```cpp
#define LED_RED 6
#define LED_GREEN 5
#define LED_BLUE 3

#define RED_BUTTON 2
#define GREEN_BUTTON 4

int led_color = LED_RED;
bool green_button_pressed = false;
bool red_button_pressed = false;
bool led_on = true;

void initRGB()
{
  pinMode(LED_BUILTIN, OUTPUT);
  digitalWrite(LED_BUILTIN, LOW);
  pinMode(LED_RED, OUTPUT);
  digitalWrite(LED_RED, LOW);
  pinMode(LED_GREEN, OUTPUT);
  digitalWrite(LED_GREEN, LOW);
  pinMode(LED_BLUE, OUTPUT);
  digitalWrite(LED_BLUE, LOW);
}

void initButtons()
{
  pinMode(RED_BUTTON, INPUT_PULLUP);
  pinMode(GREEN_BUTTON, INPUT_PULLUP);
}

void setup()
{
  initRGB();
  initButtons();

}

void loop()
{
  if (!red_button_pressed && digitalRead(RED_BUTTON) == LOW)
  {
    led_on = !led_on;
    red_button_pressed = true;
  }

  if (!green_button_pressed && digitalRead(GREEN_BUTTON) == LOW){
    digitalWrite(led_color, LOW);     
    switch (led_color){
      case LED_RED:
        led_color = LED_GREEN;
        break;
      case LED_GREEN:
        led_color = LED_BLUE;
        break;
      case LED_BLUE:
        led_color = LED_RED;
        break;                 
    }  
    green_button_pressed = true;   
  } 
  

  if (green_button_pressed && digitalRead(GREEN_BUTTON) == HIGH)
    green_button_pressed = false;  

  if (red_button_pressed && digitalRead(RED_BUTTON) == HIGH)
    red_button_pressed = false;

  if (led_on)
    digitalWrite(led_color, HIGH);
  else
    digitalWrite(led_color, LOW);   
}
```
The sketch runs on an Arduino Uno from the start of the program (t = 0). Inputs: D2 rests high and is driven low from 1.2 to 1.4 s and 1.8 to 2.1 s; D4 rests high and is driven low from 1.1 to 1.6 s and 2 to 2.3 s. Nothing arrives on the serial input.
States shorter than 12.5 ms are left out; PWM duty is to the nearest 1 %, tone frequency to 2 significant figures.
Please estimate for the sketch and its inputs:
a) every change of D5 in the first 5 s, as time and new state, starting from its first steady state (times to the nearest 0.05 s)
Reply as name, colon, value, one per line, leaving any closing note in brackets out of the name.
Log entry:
every change of D5 in the first 5 s, as time and new state, starting from its first steady state: 0 s low; 1.1 s high; 1.2 s low; 1.8 s high; 2 s low
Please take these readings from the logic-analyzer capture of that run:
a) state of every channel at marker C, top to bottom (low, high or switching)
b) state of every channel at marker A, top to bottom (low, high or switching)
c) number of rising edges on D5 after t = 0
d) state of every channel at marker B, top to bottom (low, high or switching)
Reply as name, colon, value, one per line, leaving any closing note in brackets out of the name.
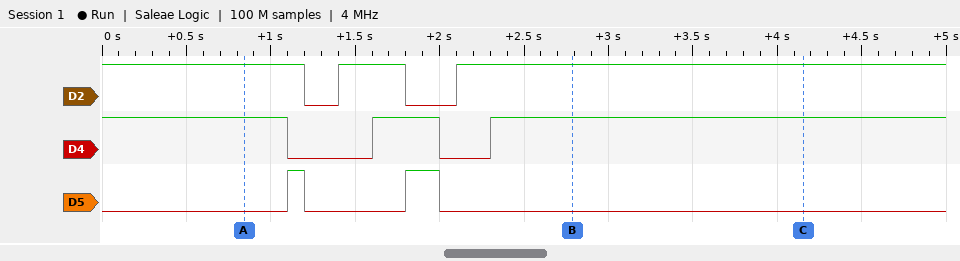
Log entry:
state of every channel at marker C, top to bottom: D2 high, D4 high, D5 low
state of every channel at marker A, top to bottom: D2 high, D4 high, D5 low
number of rising edges on D5 after t = 0: 2
state of every channel at marker B, top to bottom: D2 high, D4 high, D5 low
